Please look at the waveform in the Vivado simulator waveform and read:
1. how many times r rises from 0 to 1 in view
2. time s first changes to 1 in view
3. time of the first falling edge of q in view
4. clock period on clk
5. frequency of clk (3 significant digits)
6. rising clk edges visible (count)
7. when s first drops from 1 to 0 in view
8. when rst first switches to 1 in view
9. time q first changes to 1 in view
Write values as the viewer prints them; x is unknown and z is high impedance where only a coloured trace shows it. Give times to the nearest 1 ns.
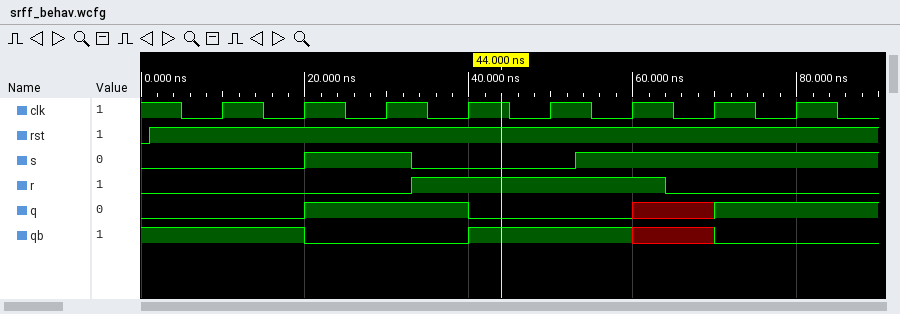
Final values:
1
20 ns
40 ns
10 ns
100 MHz
8
33 ns
1 ns
20 ns
